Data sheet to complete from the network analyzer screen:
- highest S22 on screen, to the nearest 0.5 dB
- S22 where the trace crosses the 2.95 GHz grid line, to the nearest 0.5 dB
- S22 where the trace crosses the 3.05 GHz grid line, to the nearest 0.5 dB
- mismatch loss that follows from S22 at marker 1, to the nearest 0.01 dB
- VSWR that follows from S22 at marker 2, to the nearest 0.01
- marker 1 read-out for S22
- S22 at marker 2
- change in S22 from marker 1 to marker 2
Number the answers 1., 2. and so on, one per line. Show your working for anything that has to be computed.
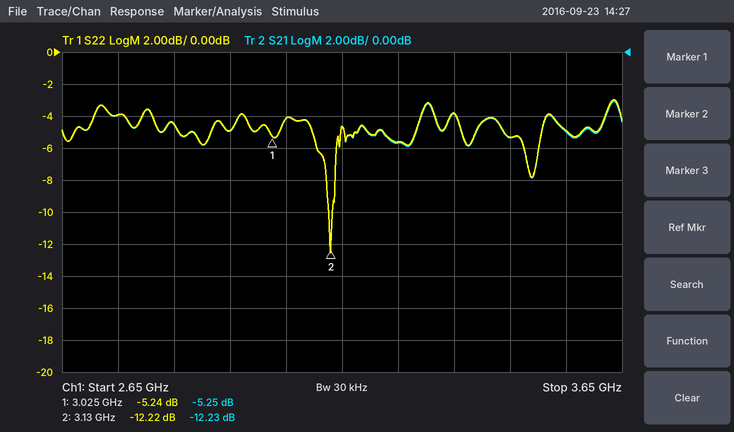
1. -3.0 dB
2. -5.0 dB
3. -4.0 dB
4. −10 log10(1 − 10^(-5.24/10)) ≈ 1.54 dB
5. (1 + 0.2449)/(1 − 0.2449) ≈ 1.65
6. -5.24 dB
7. -12.22 dB
8. -12.22 − (-5.24) = -6.98 dB
